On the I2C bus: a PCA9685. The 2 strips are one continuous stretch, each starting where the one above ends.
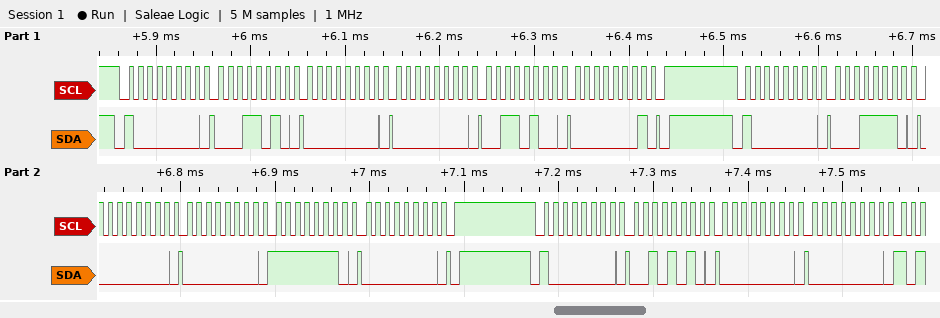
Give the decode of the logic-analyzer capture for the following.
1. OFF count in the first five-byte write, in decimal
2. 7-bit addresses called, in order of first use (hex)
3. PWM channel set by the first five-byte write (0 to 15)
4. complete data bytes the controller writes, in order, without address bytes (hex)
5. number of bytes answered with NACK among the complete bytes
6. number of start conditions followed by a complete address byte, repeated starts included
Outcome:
308
0x40
5
1A 00 00 34 01 1E 00 00 FE 00 2A 00 00
0
3
